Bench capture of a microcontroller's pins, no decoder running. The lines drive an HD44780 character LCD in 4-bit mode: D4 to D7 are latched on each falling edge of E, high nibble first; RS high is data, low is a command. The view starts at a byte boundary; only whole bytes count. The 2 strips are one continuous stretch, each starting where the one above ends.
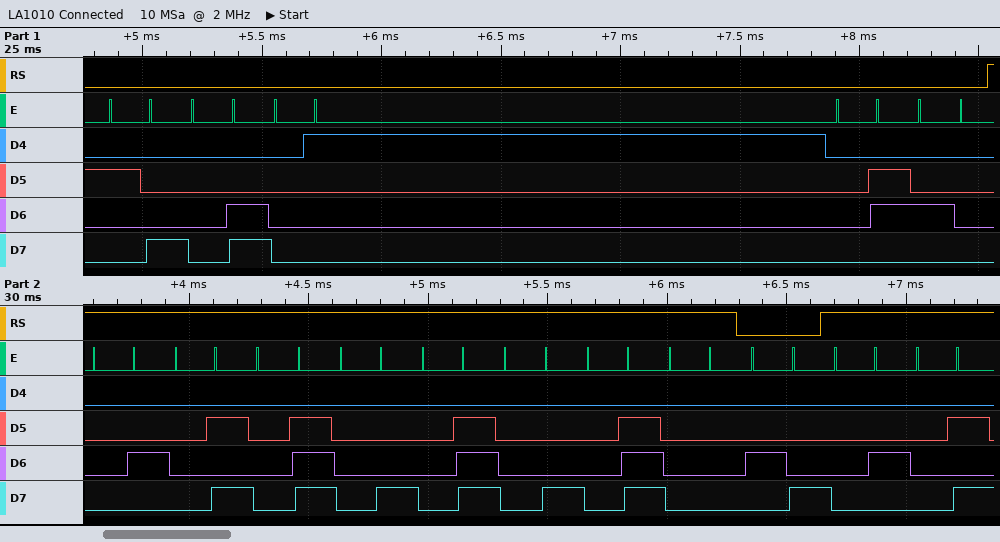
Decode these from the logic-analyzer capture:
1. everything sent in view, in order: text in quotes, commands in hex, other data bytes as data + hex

0x28 0x0C 0x01 0x06 0x40 data 04 0A 0E 08 0E 08 0E 00 0x48 data 04 0A
